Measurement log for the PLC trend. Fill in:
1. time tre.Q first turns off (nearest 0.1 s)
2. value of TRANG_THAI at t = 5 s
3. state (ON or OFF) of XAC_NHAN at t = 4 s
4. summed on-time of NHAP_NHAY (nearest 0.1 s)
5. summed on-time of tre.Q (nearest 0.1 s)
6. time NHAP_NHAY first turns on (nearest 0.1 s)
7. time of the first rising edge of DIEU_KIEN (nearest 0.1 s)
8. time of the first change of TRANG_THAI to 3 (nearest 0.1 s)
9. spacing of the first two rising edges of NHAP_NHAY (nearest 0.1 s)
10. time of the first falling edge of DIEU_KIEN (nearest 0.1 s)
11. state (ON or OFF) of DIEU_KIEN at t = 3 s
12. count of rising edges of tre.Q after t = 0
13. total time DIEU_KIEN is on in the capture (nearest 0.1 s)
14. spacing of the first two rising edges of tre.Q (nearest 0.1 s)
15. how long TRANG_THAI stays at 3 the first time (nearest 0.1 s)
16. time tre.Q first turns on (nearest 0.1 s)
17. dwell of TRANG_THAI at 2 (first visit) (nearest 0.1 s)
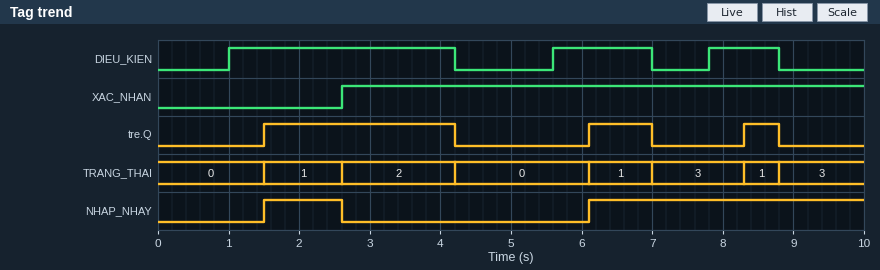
4.2 s
0
ON
5.0 s
4.1 s
1.5 s
1.0 s
7.0 s
4.6 s
4.2 s
ON
3
5.6 s
4.6 s
1.3 s
1.5 s
1.6 s
